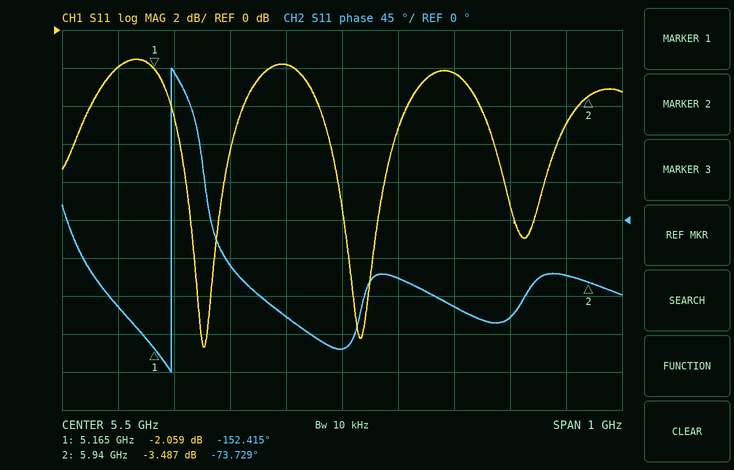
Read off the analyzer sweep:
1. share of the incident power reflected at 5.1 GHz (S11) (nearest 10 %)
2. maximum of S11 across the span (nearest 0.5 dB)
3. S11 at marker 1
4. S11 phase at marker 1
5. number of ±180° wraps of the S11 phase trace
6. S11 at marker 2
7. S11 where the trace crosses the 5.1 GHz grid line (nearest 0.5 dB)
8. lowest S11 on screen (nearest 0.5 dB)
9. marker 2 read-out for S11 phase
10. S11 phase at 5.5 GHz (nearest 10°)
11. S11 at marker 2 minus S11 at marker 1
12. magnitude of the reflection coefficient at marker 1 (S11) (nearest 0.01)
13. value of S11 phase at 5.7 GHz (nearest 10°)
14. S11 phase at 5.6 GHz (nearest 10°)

60 %
-1.5 dB
-2.059 dB
-152.415°
1
-3.487 dB
-2.0 dB
-16.5 dB
-73.729°
-150°
-1.428 dB
0.79
-100°
-70°
